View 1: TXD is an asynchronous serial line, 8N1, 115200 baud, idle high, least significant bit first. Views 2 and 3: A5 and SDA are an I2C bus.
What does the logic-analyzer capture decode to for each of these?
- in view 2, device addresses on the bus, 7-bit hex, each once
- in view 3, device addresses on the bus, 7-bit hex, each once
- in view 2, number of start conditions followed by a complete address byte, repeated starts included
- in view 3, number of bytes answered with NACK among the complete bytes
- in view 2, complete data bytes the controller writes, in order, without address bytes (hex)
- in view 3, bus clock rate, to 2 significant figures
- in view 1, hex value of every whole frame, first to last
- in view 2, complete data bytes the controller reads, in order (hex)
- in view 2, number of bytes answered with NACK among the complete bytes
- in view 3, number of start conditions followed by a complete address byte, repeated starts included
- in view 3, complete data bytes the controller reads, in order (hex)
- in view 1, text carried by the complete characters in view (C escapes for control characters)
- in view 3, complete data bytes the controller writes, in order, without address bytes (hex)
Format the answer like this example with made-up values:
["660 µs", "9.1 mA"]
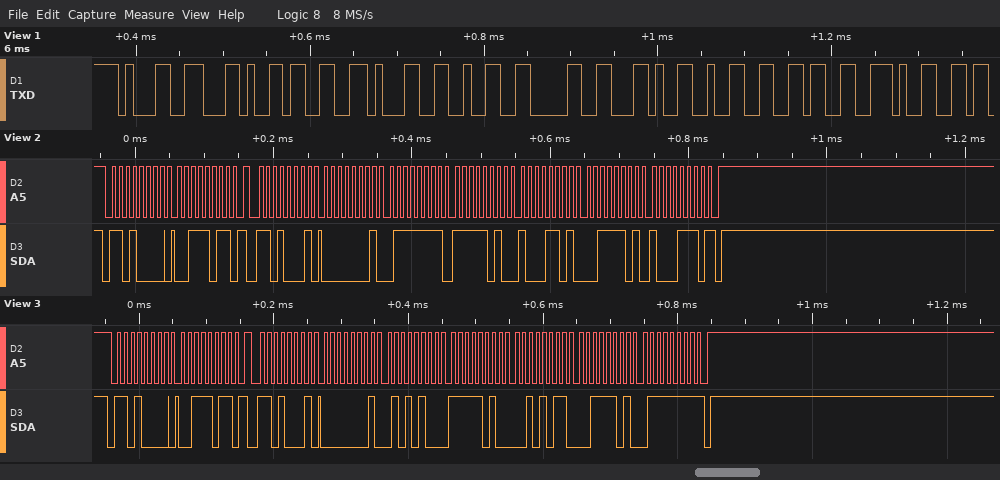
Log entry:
["0x68", "0x68", "2", "1", "3B", "100 kHz", "31 2C 33 31 32 30 2C 32 36 2E", "01 7F FA 8D 3D 8E", "1", "2", "01 54 FA 2B 3D 7F", "\"1,3120,26.\"", "3B"]
